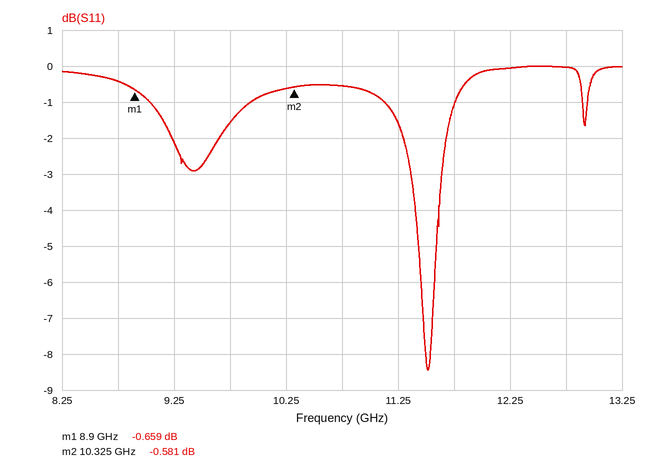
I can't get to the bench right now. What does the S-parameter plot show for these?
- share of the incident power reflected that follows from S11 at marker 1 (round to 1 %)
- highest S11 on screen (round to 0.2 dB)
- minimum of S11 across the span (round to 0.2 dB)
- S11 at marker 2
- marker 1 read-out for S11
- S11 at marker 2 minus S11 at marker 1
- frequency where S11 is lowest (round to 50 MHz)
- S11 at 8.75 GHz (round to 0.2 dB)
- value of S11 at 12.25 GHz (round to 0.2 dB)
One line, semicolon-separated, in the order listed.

86 %; 0.0 dB; -8.4 dB; -0.581 dB; -0.659 dB; 0.078 dB; 11.50 GHz; -0.4 dB; 0.0 dB
